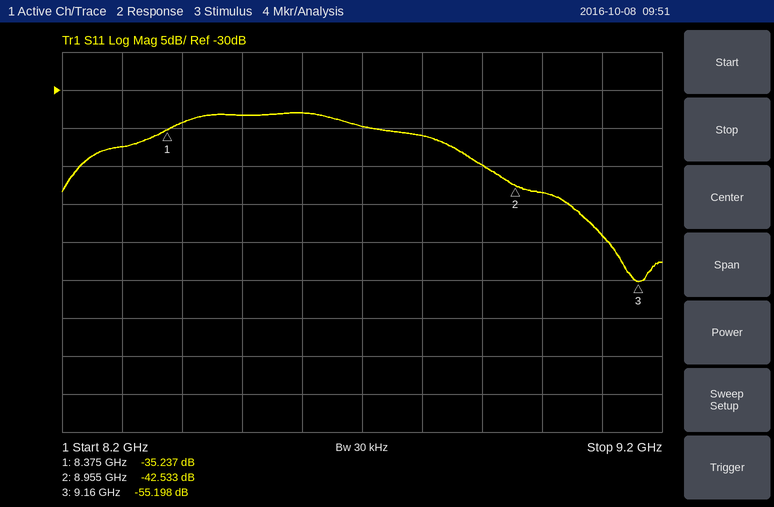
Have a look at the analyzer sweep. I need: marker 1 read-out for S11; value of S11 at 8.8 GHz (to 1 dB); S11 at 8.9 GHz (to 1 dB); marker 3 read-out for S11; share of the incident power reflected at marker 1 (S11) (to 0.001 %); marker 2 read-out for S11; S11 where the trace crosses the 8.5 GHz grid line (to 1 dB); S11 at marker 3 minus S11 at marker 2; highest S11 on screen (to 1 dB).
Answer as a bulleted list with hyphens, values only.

- -35.237 dB
- -36 dB
- -40 dB
- -55.198 dB
- 0.030 %
- -42.533 dB
- -33 dB
- -12.665 dB
- -33 dB
